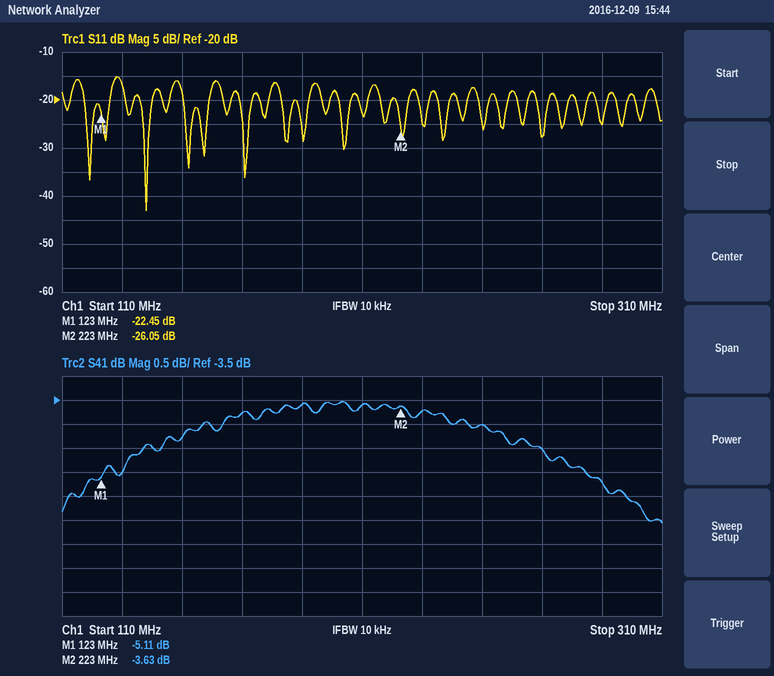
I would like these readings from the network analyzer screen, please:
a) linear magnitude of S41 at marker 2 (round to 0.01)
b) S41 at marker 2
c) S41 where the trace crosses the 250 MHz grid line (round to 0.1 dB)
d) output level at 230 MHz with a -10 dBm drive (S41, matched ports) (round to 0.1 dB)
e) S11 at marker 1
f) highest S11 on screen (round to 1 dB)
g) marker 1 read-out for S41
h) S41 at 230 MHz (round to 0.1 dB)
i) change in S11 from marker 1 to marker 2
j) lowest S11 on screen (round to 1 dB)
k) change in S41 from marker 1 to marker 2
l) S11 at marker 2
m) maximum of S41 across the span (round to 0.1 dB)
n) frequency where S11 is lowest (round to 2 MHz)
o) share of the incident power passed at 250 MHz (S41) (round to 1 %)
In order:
0.66
-3.63 dB
-4.0 dB
-13.7 dBm
-22.45 dB
-15 dB
-5.11 dB
-3.7 dB
-3.60 dB
-43 dB
1.48 dB
-26.05 dB
-3.5 dB
138 MHz
40 %
